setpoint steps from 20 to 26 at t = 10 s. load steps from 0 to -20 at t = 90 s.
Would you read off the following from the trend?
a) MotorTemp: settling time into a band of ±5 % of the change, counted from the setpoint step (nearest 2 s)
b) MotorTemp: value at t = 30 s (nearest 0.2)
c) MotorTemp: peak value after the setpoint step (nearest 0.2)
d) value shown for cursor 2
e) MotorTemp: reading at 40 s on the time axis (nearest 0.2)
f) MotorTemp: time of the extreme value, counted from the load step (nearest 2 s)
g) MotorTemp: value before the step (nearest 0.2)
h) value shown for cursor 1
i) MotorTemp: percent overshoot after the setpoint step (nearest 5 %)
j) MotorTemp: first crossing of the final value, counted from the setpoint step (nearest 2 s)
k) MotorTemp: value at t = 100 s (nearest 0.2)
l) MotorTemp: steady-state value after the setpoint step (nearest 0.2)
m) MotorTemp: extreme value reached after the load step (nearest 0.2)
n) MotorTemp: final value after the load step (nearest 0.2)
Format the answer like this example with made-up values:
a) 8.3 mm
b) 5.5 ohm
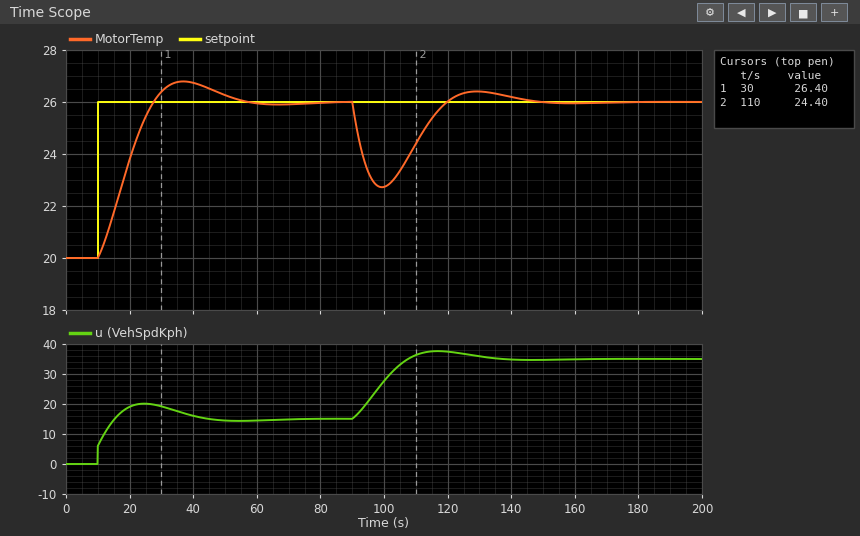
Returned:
a) 40 s
b) 26.4
c) 26.8
d) 24.40
e) 26.8
f) 10 s
g) 20.0
h) 26.40
i) 15 %
j) 18 s
k) 22.8
l) 26.0
m) 22.8
n) 26.0
